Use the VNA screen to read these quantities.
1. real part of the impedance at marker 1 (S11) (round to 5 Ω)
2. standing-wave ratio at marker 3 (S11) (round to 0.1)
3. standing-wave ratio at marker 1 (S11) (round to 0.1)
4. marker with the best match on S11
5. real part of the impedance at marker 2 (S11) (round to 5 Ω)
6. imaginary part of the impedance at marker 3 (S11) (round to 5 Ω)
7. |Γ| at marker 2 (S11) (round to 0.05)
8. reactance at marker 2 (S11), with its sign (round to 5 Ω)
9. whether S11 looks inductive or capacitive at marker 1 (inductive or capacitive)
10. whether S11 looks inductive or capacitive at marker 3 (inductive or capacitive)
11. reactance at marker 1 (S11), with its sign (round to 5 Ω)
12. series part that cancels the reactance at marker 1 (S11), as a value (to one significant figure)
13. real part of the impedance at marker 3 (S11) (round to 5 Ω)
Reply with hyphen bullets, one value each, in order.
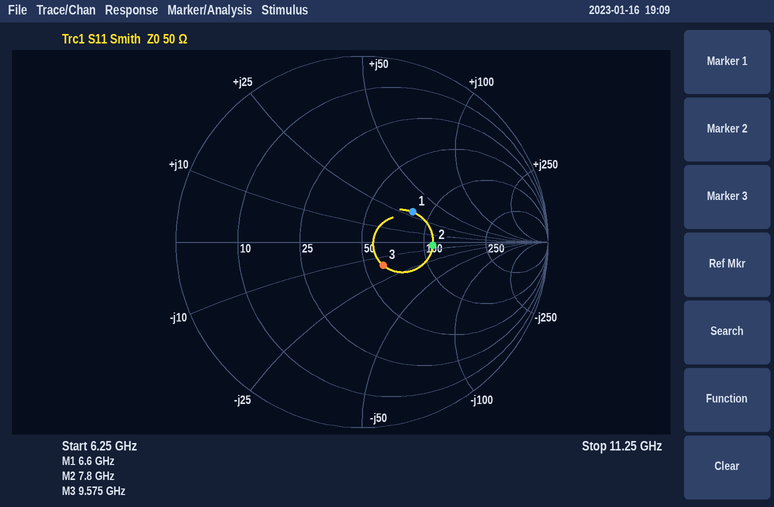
- 80 Ω
- 1.4
- 1.9
- marker 3
- 110 Ω
- -15 Ω
- 0.40
- -5 Ω
- inductive
- capacitive
- +30 Ω
- 800 fF
- 60 Ω
